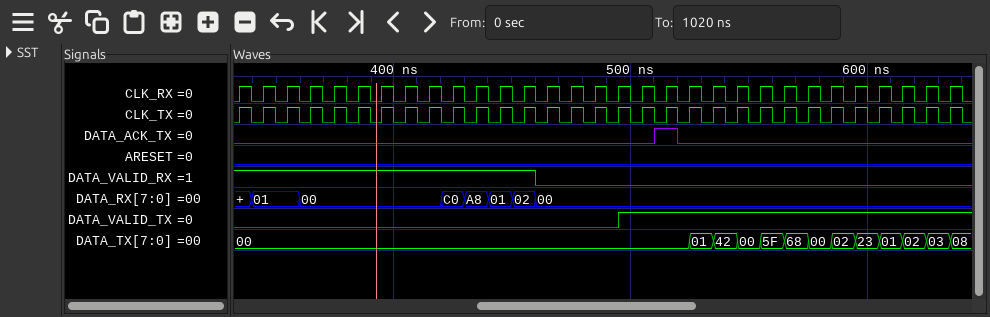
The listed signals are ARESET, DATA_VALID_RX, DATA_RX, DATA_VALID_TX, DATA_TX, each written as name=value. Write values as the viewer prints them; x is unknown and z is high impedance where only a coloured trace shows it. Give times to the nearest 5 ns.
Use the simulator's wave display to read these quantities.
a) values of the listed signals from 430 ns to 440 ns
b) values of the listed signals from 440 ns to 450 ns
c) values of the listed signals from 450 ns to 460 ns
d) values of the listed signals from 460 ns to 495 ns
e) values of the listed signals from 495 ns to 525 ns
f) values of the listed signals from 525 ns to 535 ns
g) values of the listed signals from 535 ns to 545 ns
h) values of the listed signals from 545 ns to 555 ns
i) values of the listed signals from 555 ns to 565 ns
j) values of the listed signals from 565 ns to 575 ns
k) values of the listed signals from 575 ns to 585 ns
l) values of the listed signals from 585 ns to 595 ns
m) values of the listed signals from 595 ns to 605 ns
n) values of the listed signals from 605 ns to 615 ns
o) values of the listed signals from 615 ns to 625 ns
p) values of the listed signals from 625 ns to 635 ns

ARESET=0, DATA_VALID_RX=1, DATA_RX=A8, DATA_VALID_TX=0, DATA_TX=00
ARESET=0, DATA_VALID_RX=1, DATA_RX=01, DATA_VALID_TX=0, DATA_TX=00
ARESET=0, DATA_VALID_RX=1, DATA_RX=02, DATA_VALID_TX=0, DATA_TX=00
ARESET=0, DATA_VALID_RX=0, DATA_RX=00, DATA_VALID_TX=0, DATA_TX=00
ARESET=0, DATA_VALID_RX=0, DATA_RX=00, DATA_VALID_TX=1, DATA_TX=00
ARESET=0, DATA_VALID_RX=0, DATA_RX=00, DATA_VALID_TX=1, DATA_TX=01
ARESET=0, DATA_VALID_RX=0, DATA_RX=00, DATA_VALID_TX=1, DATA_TX=42
ARESET=0, DATA_VALID_RX=0, DATA_RX=00, DATA_VALID_TX=1, DATA_TX=00
ARESET=0, DATA_VALID_RX=0, DATA_RX=00, DATA_VALID_TX=1, DATA_TX=5F
ARESET=0, DATA_VALID_RX=0, DATA_RX=00, DATA_VALID_TX=1, DATA_TX=68
ARESET=0, DATA_VALID_RX=0, DATA_RX=00, DATA_VALID_TX=1, DATA_TX=00
ARESET=0, DATA_VALID_RX=0, DATA_RX=00, DATA_VALID_TX=1, DATA_TX=02
ARESET=0, DATA_VALID_RX=0, DATA_RX=00, DATA_VALID_TX=1, DATA_TX=23
ARESET=0, DATA_VALID_RX=0, DATA_RX=00, DATA_VALID_TX=1, DATA_TX=01
ARESET=0, DATA_VALID_RX=0, DATA_RX=00, DATA_VALID_TX=1, DATA_TX=02
ARESET=0, DATA_VALID_RX=0, DATA_RX=00, DATA_VALID_TX=1, DATA_TX=03
